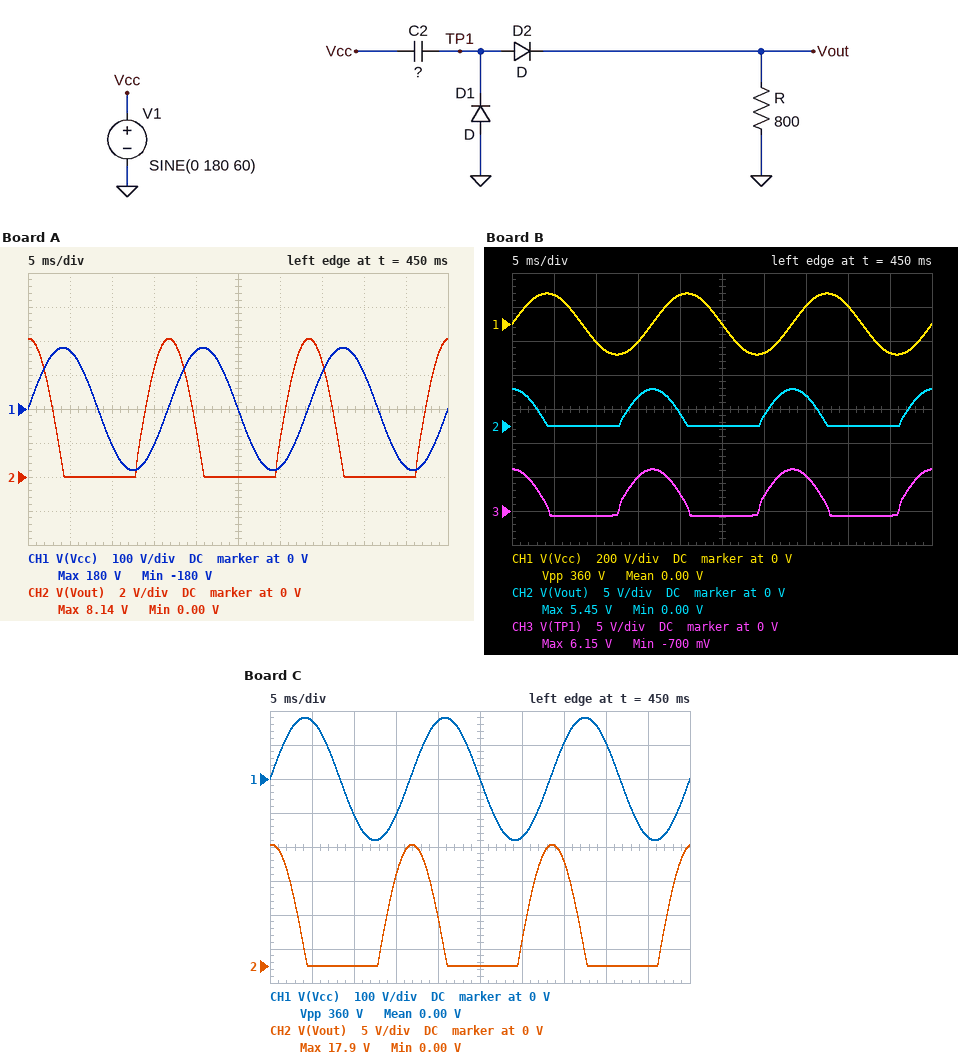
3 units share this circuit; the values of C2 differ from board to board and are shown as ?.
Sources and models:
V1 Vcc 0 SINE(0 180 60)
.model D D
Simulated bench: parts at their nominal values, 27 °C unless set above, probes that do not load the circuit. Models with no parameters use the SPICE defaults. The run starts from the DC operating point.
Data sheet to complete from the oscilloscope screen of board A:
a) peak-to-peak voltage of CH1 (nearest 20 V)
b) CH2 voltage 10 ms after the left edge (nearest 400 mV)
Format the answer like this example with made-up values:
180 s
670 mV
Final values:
360 V
0 V
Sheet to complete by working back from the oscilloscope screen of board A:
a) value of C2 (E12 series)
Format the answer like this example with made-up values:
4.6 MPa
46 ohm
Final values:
150 nF
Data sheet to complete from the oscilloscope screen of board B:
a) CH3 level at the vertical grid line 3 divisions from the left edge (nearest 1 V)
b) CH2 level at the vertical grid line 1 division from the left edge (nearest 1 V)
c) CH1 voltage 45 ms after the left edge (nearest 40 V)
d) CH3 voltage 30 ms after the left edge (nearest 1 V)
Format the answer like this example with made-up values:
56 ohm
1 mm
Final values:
5 V
0 V
-160 V
2 V
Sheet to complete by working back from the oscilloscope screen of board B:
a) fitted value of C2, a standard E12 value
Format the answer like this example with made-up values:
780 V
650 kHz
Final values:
100 nF
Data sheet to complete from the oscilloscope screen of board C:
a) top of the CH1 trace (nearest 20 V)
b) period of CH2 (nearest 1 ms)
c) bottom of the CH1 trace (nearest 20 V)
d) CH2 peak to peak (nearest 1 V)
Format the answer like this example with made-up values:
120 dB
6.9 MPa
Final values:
180 V
17 ms
-180 V
18 V
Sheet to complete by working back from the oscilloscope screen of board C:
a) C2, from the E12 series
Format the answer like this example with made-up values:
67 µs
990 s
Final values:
330 nF
